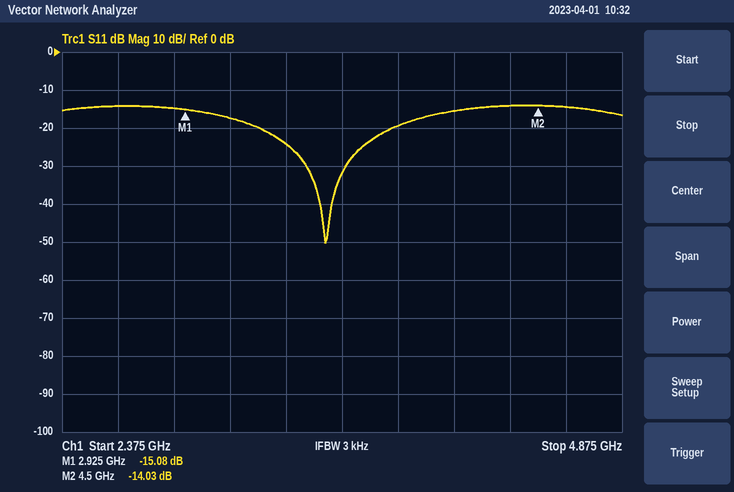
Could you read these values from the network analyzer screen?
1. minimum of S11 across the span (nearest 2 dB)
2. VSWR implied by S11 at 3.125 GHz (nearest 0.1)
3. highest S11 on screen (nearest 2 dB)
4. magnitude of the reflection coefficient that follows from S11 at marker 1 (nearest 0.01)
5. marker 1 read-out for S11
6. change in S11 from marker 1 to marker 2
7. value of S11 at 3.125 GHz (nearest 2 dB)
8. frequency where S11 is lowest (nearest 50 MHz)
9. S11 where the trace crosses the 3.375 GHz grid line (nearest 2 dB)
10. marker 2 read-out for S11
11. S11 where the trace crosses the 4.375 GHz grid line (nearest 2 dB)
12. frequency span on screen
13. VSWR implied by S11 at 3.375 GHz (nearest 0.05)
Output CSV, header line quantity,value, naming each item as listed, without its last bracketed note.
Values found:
quantity,value
minimum of S11 across the span,-50 dB
VSWR implied by S11 at 3.125 GHz,1.3
highest S11 on screen,-14 dB
magnitude of the reflection coefficient that follows from S11 at marker 1,0.18
marker 1 read-out for S11,-15.08 dB
change in S11 from marker 1 to marker 2,1.05 dB
value of S11 at 3.125 GHz,-18 dB
frequency where S11 is lowest,3.55 GHz
S11 where the trace crosses the 3.375 GHz grid line,-24 dB
marker 2 read-out for S11,-14.03 dB
S11 where the trace crosses the 4.375 GHz grid line,-14 dB
frequency span on screen,2.5 GHz
VSWR implied by S11 at 3.375 GHz,1.15
